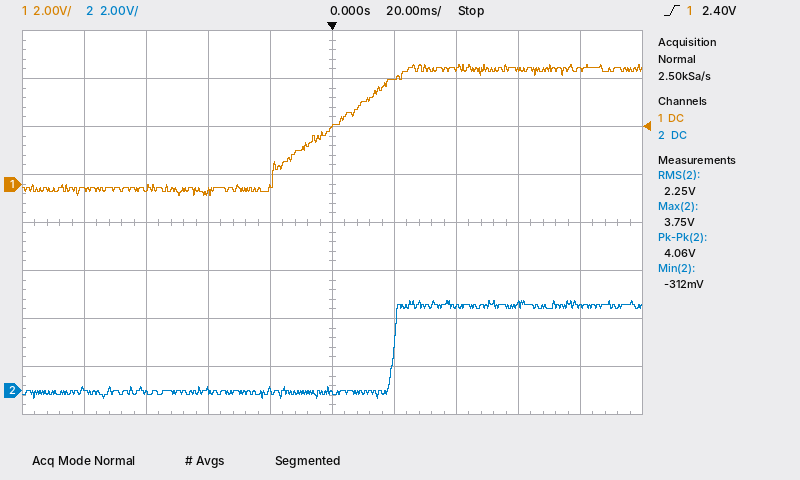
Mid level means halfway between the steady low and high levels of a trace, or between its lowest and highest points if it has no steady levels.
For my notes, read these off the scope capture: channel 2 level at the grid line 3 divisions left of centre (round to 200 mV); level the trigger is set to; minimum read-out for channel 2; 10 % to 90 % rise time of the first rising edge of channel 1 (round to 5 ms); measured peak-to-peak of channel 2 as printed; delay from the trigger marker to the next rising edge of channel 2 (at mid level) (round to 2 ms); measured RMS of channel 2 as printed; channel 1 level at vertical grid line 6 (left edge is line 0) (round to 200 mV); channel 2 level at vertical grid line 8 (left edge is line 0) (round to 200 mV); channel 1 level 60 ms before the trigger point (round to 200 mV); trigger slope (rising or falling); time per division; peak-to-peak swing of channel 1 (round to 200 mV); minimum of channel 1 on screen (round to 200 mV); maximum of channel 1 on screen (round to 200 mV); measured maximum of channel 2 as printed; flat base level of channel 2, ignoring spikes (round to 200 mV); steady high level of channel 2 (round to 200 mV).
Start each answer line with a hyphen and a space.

- 0.0 V
- 2.40 V
- -312 mV
- 35 ms
- 4.06 V
- 20 ms
- 2.25 V
- 4.4 V
- 3.6 V
- -200 mV
- rising
- 20 ms
- 5.4 V
- -400 mV
- 5.0 V
- 3.75 V
- 0.0 V
- 3.6 V
